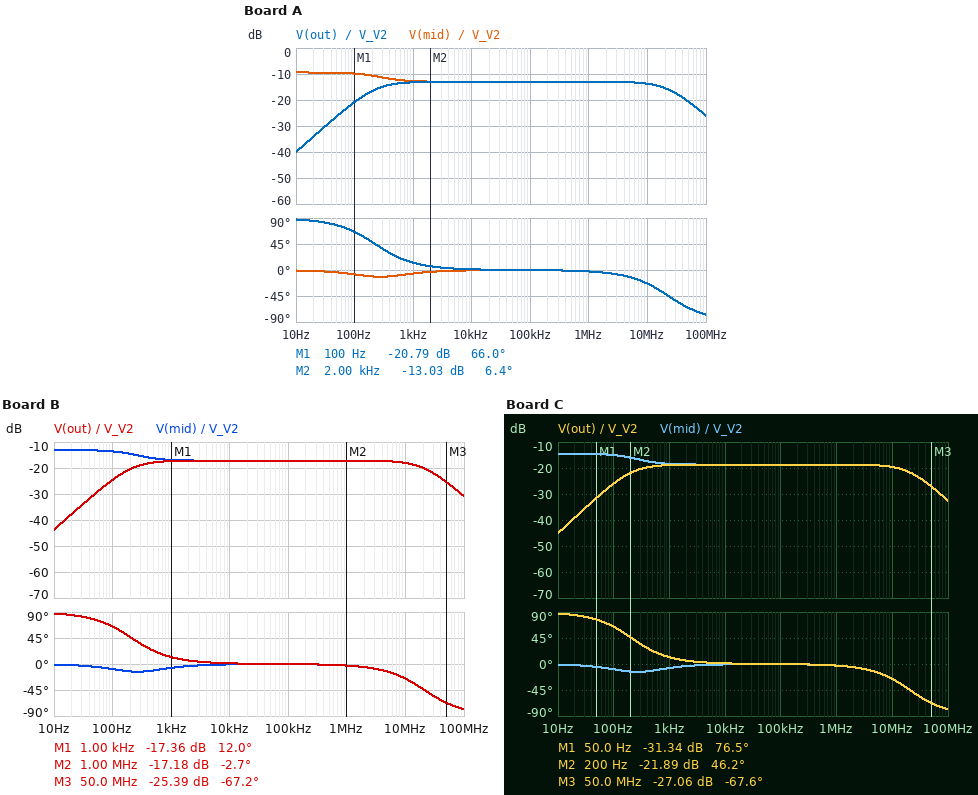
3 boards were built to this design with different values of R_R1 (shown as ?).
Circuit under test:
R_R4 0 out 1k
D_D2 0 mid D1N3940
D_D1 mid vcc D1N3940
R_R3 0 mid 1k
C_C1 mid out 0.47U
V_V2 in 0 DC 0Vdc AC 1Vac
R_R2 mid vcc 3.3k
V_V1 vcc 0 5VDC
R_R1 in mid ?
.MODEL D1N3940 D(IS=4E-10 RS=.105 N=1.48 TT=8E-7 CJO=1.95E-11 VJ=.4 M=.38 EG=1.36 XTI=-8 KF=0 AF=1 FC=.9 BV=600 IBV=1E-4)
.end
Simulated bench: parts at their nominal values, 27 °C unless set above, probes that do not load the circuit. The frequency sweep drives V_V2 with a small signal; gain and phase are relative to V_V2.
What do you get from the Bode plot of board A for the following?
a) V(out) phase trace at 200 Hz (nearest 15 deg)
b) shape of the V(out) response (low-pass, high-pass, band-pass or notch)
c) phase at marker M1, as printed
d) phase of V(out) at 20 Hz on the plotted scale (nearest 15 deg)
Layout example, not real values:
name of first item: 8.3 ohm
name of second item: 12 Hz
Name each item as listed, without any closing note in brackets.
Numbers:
V(out) phase trace at 200 Hz: 45 deg
shape of the V(out) response: band-pass
phase at marker M1, as printed: 66.0 deg
phase of V(out) at 20 Hz on the plotted scale: 90 deg
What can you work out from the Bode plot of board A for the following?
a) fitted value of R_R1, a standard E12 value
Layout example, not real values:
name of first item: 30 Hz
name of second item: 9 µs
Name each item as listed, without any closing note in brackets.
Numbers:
fitted value of R_R1, a standard E12 value: 1.5 kΩ
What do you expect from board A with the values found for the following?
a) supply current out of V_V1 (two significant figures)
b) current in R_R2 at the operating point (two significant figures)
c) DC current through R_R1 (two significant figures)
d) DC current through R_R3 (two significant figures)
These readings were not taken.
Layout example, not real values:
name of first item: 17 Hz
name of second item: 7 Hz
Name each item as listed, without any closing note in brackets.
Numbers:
supply current out of V_V1: 1.3 mA
current in R_R2 at the operating point: 1.3 mA
DC current through R_R1: 510 µA
DC current through R_R3: 770 µA
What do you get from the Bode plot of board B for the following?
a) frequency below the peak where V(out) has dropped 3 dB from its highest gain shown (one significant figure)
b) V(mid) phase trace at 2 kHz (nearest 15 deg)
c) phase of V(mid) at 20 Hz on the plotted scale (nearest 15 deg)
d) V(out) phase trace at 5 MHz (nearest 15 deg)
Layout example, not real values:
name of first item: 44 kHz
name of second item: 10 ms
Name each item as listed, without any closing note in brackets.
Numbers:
frequency below the peak where V(out) has dropped 3 dB from its highest gain shown: 200 Hz
V(mid) phase trace at 2 kHz: 0 deg
phase of V(mid) at 20 Hz on the plotted scale: 0 deg
V(out) phase trace at 5 MHz: -15 deg
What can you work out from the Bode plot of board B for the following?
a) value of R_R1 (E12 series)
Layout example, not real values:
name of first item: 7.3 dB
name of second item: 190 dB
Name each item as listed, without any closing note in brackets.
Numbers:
value of R_R1: 2.7 kΩ
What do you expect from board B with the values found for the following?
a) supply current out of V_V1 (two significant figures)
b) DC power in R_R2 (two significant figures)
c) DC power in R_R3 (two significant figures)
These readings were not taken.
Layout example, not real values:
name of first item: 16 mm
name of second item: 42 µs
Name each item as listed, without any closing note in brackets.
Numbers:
supply current out of V_V1: 1.2 mA
DC power in R_R2: 5.1 mW
DC power in R_R3: 820 µW
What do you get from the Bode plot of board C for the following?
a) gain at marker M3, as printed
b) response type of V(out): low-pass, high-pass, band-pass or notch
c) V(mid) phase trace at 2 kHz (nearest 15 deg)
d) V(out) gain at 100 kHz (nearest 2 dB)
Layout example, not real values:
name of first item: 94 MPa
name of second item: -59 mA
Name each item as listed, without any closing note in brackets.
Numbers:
gain at marker M3, as printed: -27.06 dB
response type of V(out): low-pass, high-pass, band-pass or notch: band-pass
V(mid) phase trace at 2 kHz: 0 deg
V(out) gain at 100 kHz: -18 dB
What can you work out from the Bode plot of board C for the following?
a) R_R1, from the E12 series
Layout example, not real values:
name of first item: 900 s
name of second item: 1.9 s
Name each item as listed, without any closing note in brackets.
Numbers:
R_R1, from the E12 series: 3.3 kΩ
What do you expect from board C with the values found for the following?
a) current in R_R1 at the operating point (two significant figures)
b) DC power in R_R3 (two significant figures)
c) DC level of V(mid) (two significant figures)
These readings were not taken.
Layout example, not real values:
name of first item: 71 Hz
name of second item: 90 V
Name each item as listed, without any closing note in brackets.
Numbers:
current in R_R1 at the operating point: 290 µA
DC power in R_R3: 890 µW
DC level of V(mid): 940 mV
